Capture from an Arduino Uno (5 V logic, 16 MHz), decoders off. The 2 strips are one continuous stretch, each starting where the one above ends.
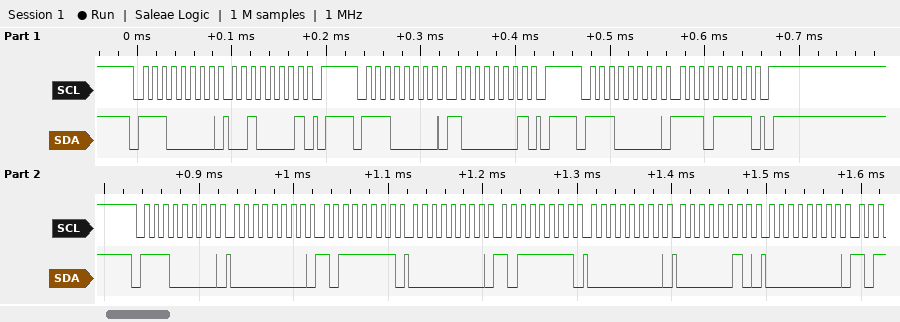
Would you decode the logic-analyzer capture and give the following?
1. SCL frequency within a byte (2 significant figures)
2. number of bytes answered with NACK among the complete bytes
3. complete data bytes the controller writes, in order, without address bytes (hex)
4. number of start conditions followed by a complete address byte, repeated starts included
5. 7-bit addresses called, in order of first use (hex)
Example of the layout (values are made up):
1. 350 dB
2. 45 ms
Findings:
1. 100 kHz
2. 0
3. 21 81 EF 00 BF 00 BF 00 02 00
4. 4
5. 0x70
